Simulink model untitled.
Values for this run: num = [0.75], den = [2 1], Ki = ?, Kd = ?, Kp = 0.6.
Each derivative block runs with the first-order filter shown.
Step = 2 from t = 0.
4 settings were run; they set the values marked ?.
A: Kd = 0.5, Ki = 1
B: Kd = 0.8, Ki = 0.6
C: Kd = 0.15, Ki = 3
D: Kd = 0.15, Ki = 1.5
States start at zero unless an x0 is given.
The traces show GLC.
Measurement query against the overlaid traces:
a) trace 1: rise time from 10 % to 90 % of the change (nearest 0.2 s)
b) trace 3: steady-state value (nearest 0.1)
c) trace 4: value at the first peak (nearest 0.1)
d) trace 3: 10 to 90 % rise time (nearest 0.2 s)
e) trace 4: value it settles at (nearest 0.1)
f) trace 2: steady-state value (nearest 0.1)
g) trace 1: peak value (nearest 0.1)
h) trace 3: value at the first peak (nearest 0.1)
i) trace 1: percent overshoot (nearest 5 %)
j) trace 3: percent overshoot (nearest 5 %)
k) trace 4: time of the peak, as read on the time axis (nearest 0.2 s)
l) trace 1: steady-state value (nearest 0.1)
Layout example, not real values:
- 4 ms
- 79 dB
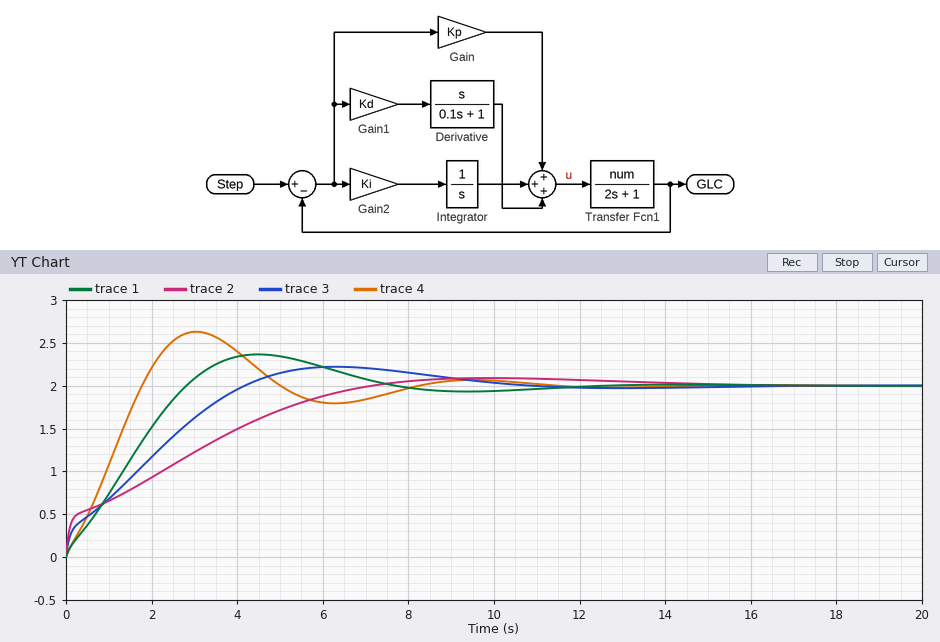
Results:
- 2.2 s
- 2.0
- 2.6
- 3.4 s
- 2.0
- 2.0
- 2.4
- 2.2
- 20 %
- 10 %
- 3.0 s
- 2.0
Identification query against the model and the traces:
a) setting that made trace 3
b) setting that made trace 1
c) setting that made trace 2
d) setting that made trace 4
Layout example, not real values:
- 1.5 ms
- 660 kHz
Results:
- A
- D
- B
- C
